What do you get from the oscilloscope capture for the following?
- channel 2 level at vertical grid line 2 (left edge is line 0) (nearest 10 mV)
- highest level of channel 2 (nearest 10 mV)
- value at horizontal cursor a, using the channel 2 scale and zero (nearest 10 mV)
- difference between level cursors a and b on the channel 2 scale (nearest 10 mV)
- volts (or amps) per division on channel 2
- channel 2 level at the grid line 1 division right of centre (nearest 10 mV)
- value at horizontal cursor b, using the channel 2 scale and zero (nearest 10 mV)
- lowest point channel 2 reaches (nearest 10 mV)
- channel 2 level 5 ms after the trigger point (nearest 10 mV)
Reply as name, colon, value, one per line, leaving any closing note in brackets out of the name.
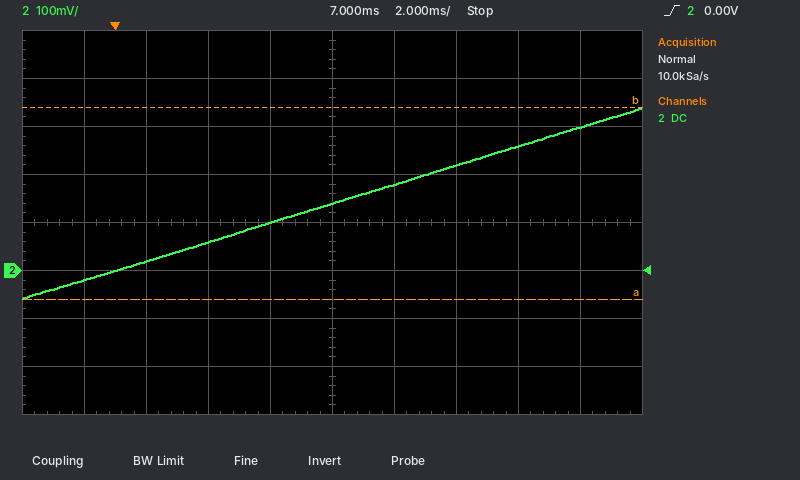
channel 2 level at vertical grid line 2 (left edge is line 0): 20 mV
highest level of channel 2: 340 mV
value at horizontal cursor a, using the channel 2 scale and zero: -60 mV
difference between level cursors a and b on the channel 2 scale: 400 mV
volts (or amps) per division on channel 2: 100 mV
channel 2 level at the grid line 1 division right of centre: 180 mV
value at horizontal cursor b, using the channel 2 scale and zero: 340 mV
lowest point channel 2 reaches: -60 mV
channel 2 level 5 ms after the trigger point: 100 mV
